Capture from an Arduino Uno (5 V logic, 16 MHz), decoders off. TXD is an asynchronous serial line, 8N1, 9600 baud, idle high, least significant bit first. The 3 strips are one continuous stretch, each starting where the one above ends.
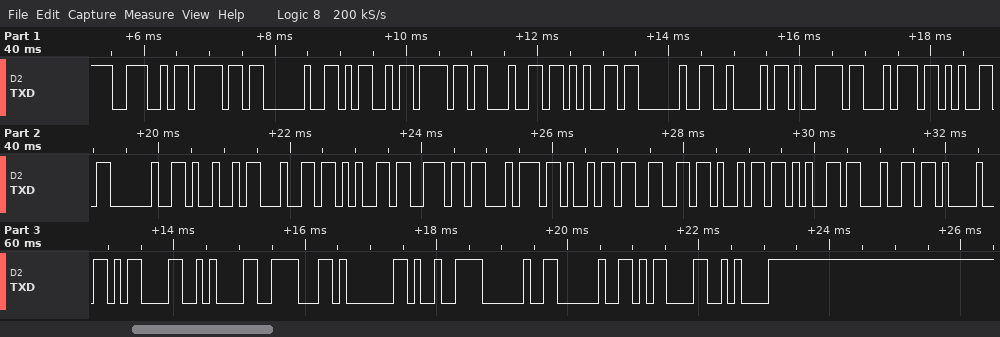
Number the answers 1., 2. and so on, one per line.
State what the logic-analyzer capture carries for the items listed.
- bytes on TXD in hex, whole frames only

1. 4E 6F 20 4D 6F 64 65 20 42 79 74 65 20 49 64 65 6E 74 69 66 69 65 64 21 0D 0A 1E 01 C9 20 20 0D 0A
